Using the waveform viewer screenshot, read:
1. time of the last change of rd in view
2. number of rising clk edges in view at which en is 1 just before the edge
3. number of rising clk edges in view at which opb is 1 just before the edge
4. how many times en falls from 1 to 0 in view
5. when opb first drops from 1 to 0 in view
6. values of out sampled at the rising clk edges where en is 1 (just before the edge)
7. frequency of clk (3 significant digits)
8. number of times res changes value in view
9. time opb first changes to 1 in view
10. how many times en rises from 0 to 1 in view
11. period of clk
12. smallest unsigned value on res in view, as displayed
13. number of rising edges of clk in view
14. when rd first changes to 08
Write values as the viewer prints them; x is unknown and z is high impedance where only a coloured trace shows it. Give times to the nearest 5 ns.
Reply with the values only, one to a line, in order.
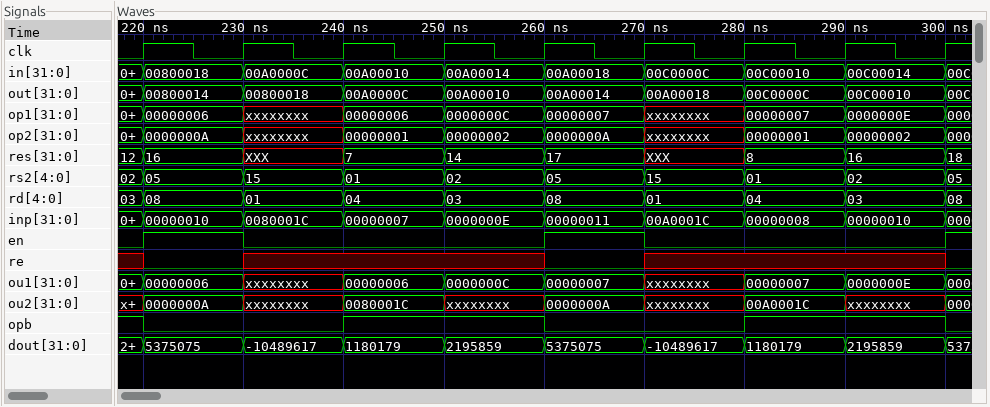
300 ns
2
5
2
220 ns
00800014, 00A00014
100 MHz
9
240 ns
3
10 ns
7
9
220 ns
